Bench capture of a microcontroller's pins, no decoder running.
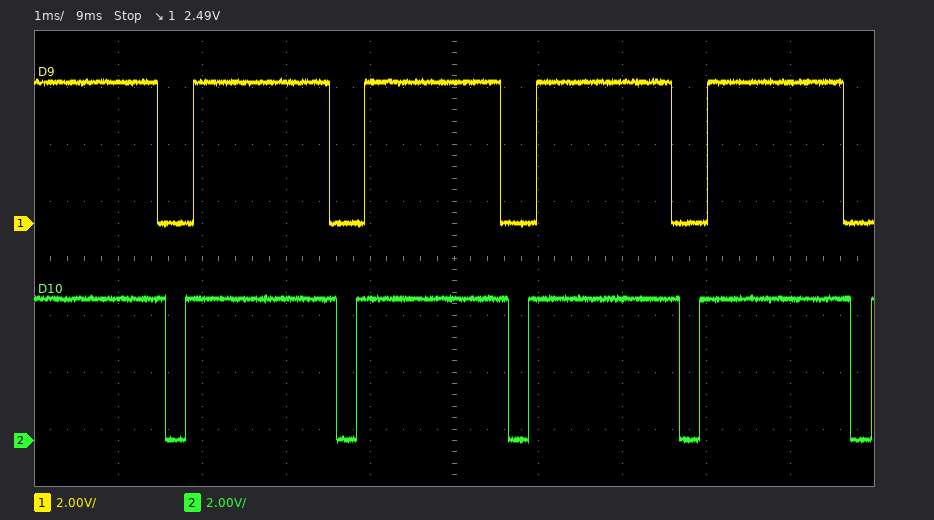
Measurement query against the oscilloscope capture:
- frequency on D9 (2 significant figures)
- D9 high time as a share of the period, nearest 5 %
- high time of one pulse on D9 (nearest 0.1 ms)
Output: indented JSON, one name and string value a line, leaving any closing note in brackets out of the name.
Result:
{
  "frequency on D9": "490 Hz",
  "D9 high time as a share of the period, nearest 5 %": "80 %",
  "high time of one pulse on D9": "1.6 ms"
}
